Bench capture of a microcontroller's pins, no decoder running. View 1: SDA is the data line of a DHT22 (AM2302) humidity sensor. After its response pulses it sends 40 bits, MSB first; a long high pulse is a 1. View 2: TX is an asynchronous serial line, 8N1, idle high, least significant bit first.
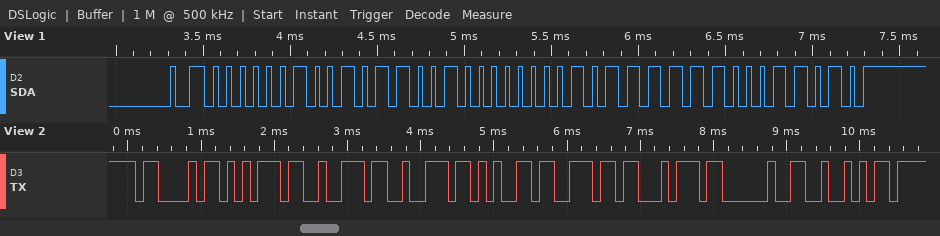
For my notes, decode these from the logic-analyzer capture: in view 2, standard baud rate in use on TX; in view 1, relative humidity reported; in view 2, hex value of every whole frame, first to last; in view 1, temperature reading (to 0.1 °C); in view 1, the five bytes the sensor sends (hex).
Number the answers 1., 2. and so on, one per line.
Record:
1. 9600 baud
2. 60.1 %
3. 43 75 72 72 65 6E 74 20 52
4. 19.1 °C
5. 02 59 00 BF 1A
